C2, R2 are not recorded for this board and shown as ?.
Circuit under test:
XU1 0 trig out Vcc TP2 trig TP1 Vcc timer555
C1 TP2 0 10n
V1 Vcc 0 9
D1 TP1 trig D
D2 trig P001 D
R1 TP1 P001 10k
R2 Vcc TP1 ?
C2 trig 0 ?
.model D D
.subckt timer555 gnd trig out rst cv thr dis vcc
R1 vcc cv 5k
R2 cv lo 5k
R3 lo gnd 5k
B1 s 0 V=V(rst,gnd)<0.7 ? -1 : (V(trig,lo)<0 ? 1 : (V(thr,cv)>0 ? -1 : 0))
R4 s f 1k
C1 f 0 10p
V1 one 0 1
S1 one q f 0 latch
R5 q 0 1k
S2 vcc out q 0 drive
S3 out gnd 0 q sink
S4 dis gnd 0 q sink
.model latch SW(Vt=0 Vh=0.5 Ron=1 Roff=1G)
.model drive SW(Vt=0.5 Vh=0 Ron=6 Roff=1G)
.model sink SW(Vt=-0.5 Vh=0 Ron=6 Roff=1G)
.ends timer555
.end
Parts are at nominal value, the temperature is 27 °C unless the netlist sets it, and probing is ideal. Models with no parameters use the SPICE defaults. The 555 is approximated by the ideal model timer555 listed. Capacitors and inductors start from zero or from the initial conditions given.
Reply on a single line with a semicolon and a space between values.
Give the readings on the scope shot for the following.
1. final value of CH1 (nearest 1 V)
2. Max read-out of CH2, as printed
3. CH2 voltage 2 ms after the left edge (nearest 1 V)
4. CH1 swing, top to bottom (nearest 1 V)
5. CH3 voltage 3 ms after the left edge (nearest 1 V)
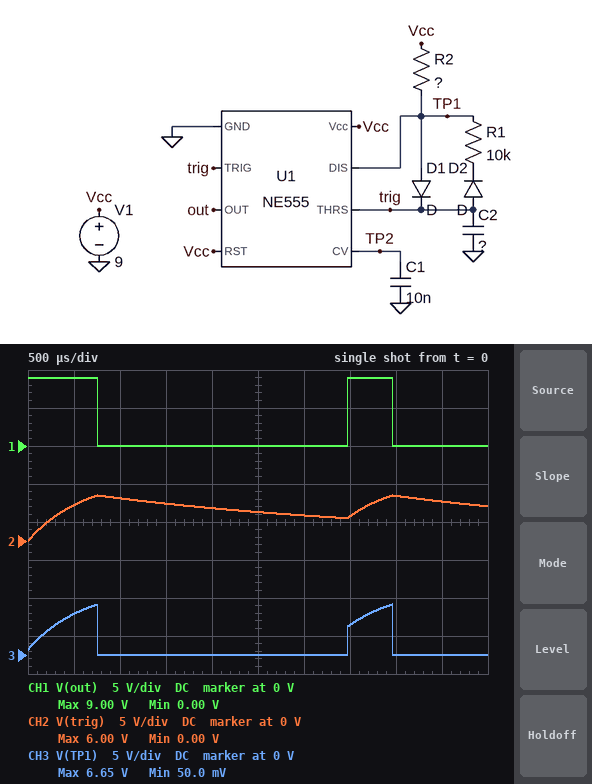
0 V; 6.00 V; 4 V; 9 V; 0 V
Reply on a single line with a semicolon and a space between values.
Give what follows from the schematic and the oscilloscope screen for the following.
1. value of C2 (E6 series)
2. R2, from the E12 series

330 nF; 1.8 kΩ
